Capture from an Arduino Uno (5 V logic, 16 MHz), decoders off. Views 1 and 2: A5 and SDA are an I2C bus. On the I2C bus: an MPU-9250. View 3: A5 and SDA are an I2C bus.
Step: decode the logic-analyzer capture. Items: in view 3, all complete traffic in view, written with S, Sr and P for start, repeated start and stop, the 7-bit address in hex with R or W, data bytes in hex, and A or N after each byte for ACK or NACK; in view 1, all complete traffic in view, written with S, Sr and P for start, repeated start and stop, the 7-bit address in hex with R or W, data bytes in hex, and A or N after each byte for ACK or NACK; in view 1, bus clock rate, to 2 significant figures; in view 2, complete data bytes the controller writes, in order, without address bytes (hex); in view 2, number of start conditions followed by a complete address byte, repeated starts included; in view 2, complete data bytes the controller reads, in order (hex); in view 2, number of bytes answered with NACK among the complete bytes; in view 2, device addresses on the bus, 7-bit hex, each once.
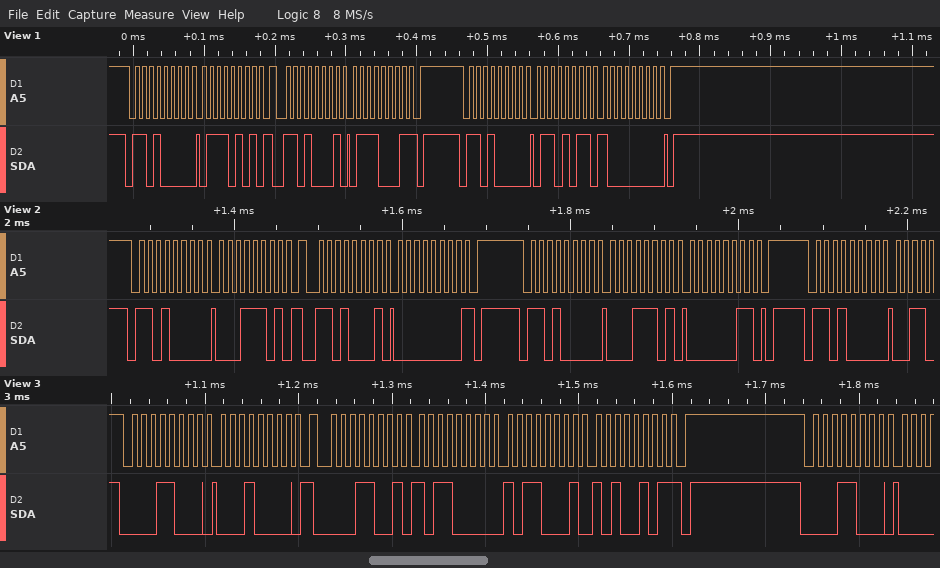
S 0CW A 10 A Sr 0CR A B0 A B1 A A5 N P S 0CW A
S 68W A 75 A Sr 68R A 71 N P S 68W A 6B A 80 A P
100 kHz
1D 1D 03
4
00
1
0x68
